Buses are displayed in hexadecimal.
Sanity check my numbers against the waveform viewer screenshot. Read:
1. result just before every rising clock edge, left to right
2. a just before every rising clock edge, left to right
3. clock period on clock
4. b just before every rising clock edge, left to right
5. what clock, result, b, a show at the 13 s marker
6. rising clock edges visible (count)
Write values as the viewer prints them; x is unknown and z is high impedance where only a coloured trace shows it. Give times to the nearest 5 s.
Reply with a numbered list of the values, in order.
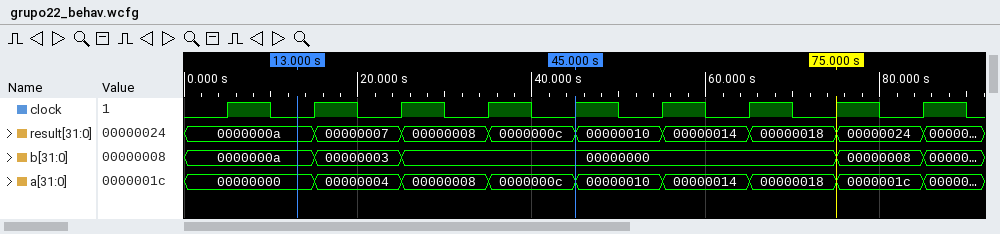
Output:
1. 0000000a, 0000000a, 00000007, 00000008, 0000000c, 00000010, 00000014, 00000018, 00000024
2. 00000000, 00000000, 00000004, 00000008, 0000000c, 00000010, 00000014, 00000018, 0000001c
3. 10 s
4. 0000000a, 0000000a, 00000003, 00000000, 00000000, 00000000, 00000000, 00000000, 00000008
5. clock=0, result=0000000a, b=0000000a, a=00000000
6. 9
